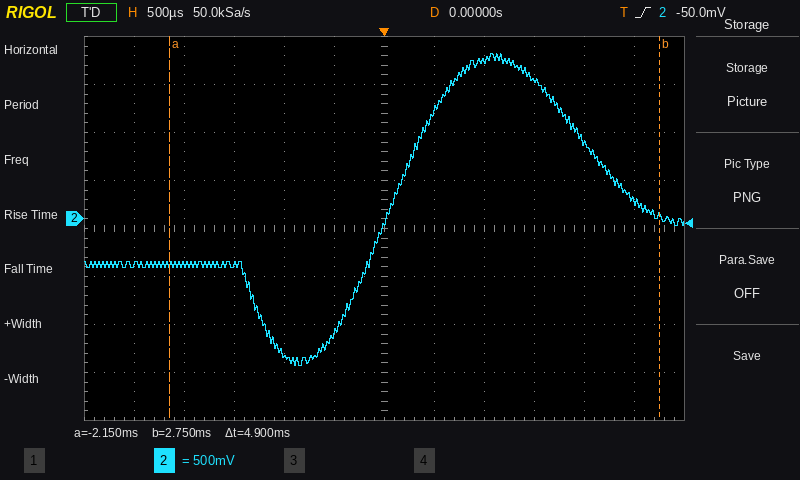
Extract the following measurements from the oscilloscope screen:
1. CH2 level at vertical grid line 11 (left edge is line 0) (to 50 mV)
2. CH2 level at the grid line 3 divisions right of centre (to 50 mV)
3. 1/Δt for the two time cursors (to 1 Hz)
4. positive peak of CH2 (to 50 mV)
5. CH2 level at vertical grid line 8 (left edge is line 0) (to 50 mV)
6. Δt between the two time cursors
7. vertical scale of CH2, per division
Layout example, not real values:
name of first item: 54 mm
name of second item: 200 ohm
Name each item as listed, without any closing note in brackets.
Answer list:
CH2 level at vertical grid line 11 (left edge is line 0): 200 mV
CH2 level at the grid line 3 divisions right of centre: 1.45 V
1/Δt for the two time cursors: 204 Hz
positive peak of CH2: 1.70 V
CH2 level at vertical grid line 8 (left edge is line 0): 1.65 V
Δt between the two time cursors: 4.9 ms
vertical scale of CH2, per division: 500 mV
